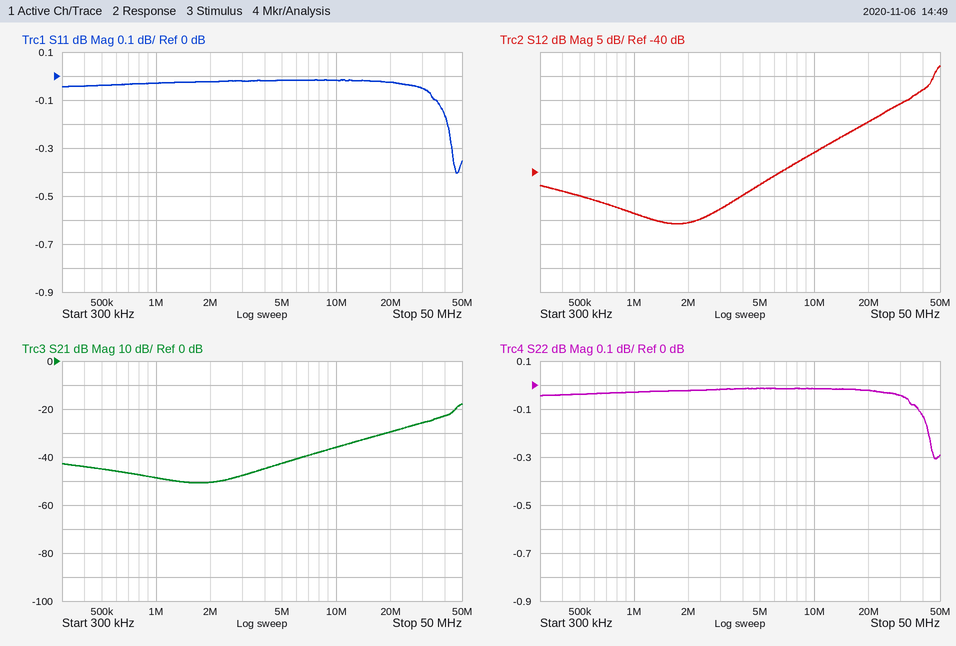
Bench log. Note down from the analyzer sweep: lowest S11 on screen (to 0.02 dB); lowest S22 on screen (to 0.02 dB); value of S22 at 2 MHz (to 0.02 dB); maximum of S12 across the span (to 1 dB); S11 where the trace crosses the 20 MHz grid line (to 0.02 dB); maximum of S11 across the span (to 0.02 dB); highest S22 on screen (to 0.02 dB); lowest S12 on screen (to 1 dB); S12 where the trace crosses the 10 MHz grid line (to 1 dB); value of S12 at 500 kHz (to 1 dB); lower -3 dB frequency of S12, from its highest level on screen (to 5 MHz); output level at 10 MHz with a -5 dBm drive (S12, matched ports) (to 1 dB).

-0.40 dB
-0.30 dB
-0.02 dB
-18 dB
-0.02 dB
-0.02 dB
-0.02 dB
-51 dB
-36 dB
-45 dB
45 MHz
-41 dBm
